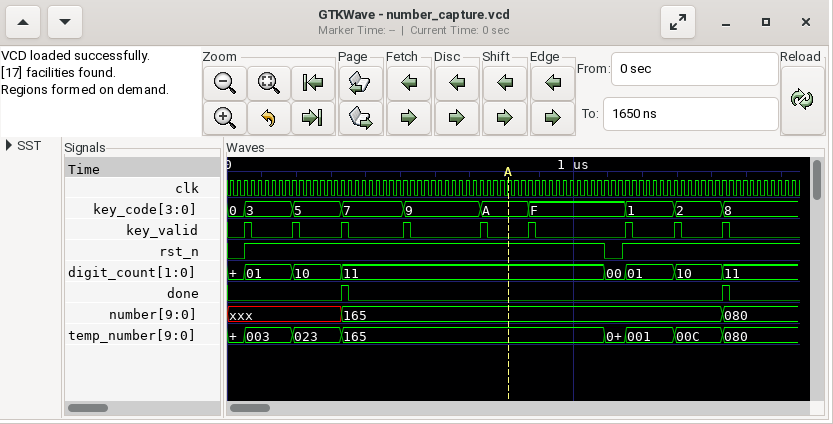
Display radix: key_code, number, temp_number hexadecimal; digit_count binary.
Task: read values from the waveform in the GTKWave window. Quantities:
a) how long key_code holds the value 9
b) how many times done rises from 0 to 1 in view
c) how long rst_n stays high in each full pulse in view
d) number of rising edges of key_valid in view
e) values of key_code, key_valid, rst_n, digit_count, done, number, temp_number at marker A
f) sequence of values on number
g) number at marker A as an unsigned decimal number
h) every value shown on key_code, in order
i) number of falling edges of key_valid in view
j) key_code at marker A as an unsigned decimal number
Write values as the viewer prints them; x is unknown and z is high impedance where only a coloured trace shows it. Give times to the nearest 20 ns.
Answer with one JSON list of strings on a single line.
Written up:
["220 ns", "2", "1040 ns", "9", "key_code=A, key_valid=0, rst_n=1, digit_count=11, done=0, number=165, temp_number=165", "xxx, 165, 080", "357", "0, 3, 5, 7, 9, A, F, 1, 2, 8", "9", "10"]
